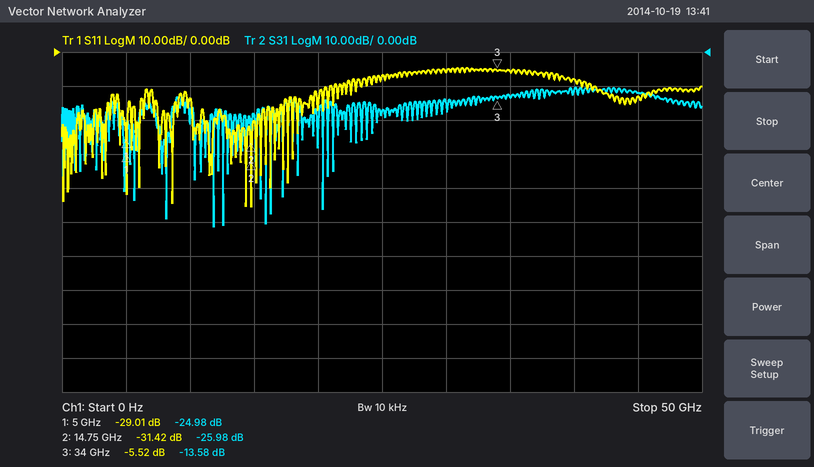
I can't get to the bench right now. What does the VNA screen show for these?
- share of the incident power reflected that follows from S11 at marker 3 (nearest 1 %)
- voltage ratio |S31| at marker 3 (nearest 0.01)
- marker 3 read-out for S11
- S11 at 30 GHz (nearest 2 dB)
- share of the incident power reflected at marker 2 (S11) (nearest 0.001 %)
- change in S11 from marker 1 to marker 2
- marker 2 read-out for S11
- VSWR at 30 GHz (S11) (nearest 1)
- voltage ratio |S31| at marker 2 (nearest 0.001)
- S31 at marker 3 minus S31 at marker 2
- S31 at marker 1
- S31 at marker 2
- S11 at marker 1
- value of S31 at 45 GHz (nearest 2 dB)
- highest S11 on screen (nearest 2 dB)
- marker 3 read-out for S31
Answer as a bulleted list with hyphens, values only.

- 28 %
- 0.21
- -5.52 dB
- -6 dB
- 0.072 %
- -2.41 dB
- -31.42 dB
- 3
- 0.050
- 12.40 dB
- -24.98 dB
- -25.98 dB
- -29.01 dB
- -12 dB
- -4 dB
- -13.58 dB
